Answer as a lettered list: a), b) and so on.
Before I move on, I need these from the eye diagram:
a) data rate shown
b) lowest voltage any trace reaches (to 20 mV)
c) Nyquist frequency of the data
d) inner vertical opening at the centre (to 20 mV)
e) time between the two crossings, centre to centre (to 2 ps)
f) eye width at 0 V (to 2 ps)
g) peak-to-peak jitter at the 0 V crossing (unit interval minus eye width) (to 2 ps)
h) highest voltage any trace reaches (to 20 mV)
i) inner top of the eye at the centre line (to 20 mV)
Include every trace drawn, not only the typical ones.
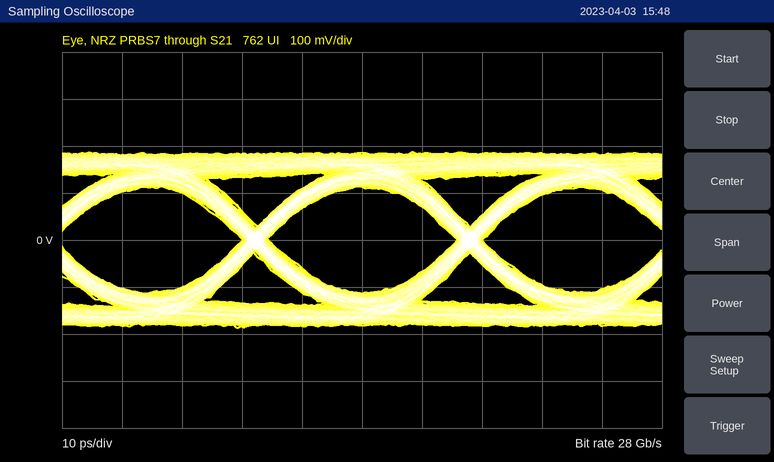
a) 28 Gb/s
b) -180 mV
c) 14 GHz
d) 220 mV
e) 36 ps
f) 32 ps
g) 4 ps
h) 180 mV
i) 120 mV
